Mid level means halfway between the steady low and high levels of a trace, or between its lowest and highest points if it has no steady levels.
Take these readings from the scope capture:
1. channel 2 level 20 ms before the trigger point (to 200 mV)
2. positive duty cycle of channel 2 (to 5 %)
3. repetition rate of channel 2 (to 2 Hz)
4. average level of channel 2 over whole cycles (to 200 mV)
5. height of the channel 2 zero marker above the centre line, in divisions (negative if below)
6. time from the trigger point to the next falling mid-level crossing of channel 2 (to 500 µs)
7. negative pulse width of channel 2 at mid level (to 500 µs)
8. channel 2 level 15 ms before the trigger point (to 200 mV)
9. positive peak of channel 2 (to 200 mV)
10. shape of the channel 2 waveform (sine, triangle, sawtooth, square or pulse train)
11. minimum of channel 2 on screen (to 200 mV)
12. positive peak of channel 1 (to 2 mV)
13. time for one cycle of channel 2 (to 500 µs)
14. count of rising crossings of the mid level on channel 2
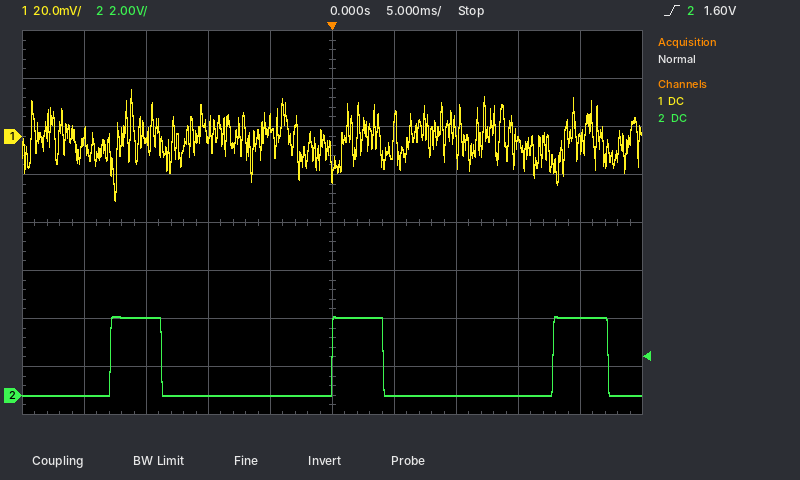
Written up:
0.0 V
25 %
56 Hz
800 mV
-3.6 div
4.0 ms
13.5 ms
3.2 V
3.2 V
pulse train
0.0 V
20 mV
18.0 ms
3
